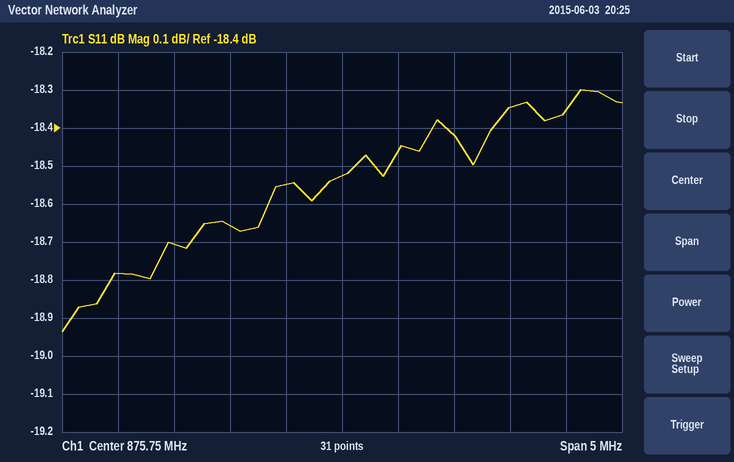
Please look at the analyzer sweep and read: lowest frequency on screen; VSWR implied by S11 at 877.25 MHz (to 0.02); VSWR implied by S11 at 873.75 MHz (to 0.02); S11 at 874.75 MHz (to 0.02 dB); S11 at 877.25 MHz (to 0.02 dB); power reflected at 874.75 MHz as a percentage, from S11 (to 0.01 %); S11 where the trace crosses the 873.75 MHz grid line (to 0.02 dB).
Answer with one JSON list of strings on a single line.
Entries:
["873.25 MHz", "1.28", "1.26", "-18.66 dB", "-18.34 dB", "1.36 %", "-18.78 dB"]
